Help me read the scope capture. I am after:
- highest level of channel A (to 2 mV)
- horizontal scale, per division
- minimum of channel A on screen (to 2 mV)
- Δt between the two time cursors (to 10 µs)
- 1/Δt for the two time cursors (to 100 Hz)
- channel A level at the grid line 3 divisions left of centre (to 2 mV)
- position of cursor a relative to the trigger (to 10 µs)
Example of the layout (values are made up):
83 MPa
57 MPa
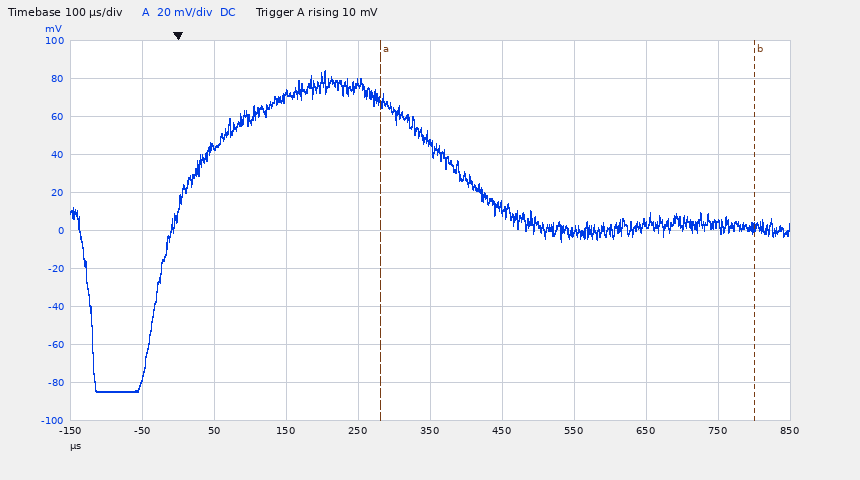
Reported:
84 mV
100 µs
-84 mV
520 µs
1.9 kHz
44 mV
+280 µs
